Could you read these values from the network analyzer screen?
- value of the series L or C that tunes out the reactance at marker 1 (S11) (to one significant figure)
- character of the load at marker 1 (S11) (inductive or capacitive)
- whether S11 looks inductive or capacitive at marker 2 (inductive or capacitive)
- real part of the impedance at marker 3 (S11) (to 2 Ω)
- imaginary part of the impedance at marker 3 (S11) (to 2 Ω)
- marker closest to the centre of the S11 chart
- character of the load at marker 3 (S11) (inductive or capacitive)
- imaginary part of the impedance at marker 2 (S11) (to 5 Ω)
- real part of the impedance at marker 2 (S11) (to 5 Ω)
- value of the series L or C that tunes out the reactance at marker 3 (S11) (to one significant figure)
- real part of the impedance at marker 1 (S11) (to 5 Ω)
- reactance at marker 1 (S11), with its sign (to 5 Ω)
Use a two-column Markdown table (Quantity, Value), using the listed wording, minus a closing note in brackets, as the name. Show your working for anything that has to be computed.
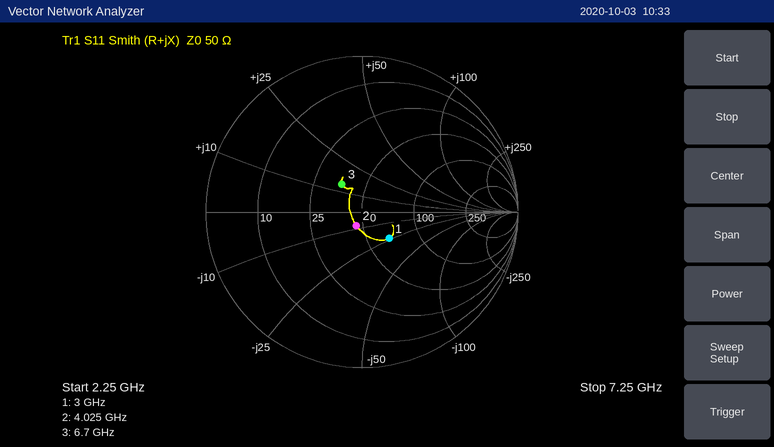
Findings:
| Quantity | Value |
|---|---|
| value of the series L or C that tunes out the reactance at marker 1 (S11) | L = 25 Ω/(2π × 3 GHz) ≈ 1 nH |
| character of the load at marker 1 (S11) | capacitive |
| whether S11 looks inductive or capacitive at marker 2 | capacitive |
| real part of the impedance at marker 3 (S11) | 36 Ω |
| imaginary part of the impedance at marker 3 (S11) | +14 Ω |
| marker closest to the centre of the S11 chart | marker 2 |
| character of the load at marker 3 (S11) | inductive |
| imaginary part of the impedance at marker 2 (S11) | -10 Ω |
| real part of the impedance at marker 2 (S11) | 45 Ω |
| value of the series L or C that tunes out the reactance at marker 3 (S11) | C = 1/(2π × 6.7 GHz × 14 Ω) ≈ 2 pF |
| real part of the impedance at marker 1 (S11) | 65 Ω |
| reactance at marker 1 (S11), with its sign | -25 Ω |
